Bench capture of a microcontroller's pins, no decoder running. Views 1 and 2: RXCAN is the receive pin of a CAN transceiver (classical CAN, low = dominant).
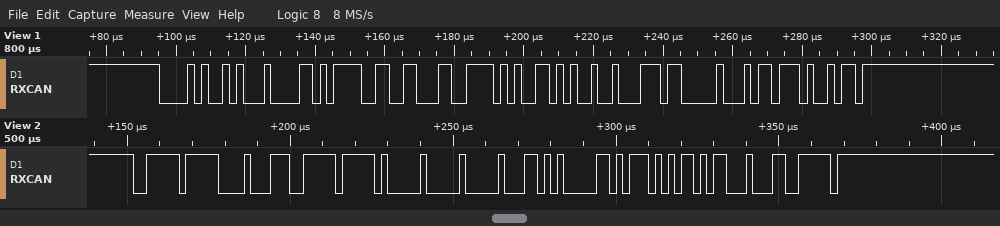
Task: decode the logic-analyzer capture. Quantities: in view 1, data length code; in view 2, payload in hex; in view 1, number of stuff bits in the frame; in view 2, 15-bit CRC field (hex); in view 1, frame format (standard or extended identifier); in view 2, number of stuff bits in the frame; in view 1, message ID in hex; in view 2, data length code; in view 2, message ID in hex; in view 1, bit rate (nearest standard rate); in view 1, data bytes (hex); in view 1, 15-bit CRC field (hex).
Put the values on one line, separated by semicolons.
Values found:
8; E7 FF 00 00 35 05 75 6B; 1; 0x08CF; standard; 8; 0x0A5; 8; 0x3FF; 500 kbit/s; 6B CC C6 7A 9A 92 3B 00; 0x5BA5
